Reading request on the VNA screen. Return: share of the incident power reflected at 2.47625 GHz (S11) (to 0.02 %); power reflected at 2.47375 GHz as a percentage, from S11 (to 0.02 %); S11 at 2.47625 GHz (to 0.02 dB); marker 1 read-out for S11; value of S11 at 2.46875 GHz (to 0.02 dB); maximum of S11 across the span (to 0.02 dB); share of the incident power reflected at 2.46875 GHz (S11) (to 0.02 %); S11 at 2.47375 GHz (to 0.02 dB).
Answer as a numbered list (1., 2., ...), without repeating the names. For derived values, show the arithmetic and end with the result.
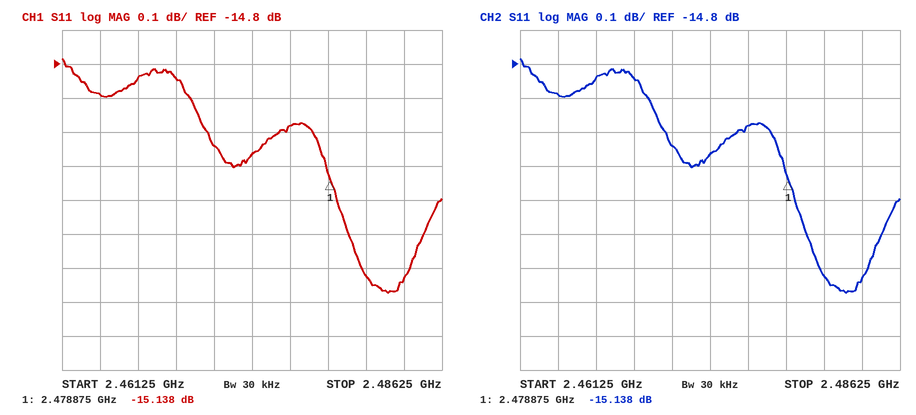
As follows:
1. 10^(-14.98/10) ≈ 3.18 %
2. 10^(-15.06/10) ≈ 3.12 %
3. -14.98 dB
4. -15.138 dB
5. -14.84 dB
6. -14.78 dB
7. 10^(-14.84/10) ≈ 3.28 %
8. -15.06 dB
